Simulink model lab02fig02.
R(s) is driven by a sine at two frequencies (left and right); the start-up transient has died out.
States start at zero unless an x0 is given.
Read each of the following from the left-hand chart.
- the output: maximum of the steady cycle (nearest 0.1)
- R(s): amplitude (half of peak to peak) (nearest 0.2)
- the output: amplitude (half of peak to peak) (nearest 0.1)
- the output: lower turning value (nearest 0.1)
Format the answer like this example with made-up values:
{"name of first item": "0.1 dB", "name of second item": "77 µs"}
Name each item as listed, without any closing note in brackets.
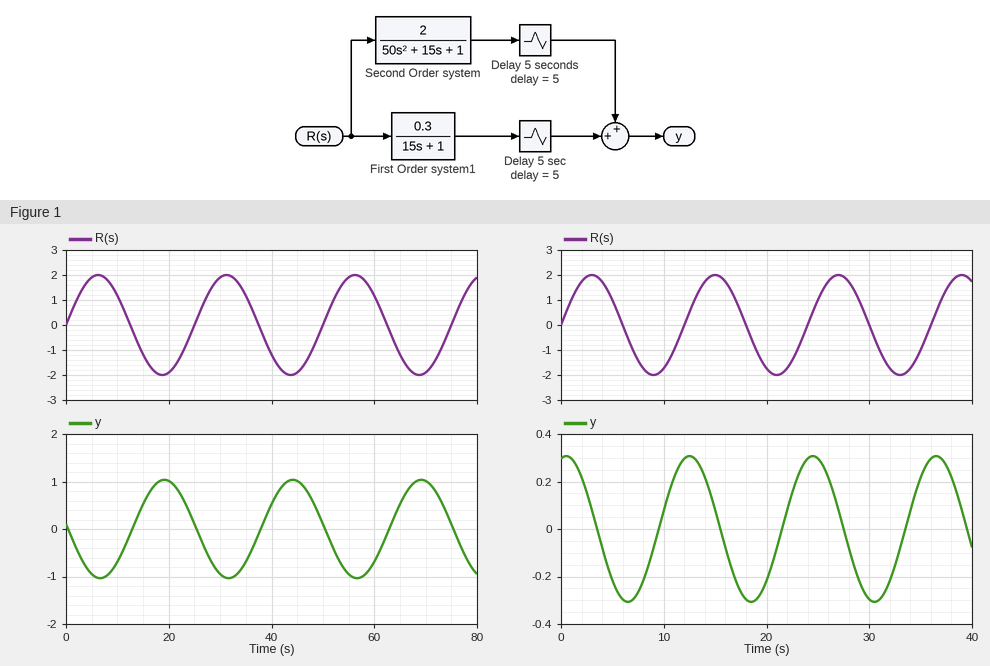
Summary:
{"the output: maximum of the steady cycle": "1.0", "R(s): amplitude (half of peak to peak)": "2.0", "the output: amplitude (half of peak to peak)": "1.0", "the output: lower turning value": "-1.0"}
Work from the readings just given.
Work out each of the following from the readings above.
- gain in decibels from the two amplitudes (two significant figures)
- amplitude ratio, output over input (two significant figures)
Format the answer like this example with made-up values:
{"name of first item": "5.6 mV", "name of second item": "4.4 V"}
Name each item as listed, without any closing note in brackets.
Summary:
{"gain in decibels from the two amplitudes": "-6.0 dB", "amplitude ratio, output over input": "0.50"}
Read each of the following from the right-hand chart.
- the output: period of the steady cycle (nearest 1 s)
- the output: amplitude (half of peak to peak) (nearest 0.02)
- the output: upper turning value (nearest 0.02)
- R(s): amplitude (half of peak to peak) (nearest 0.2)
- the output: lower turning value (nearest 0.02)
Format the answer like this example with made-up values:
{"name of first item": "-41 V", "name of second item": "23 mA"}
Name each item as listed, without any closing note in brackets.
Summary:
{"the output: period of the steady cycle": "12 s", "the output: amplitude (half of peak to peak)": "0.30", "the output: upper turning value": "0.30", "R(s): amplitude (half of peak to peak)": "2.0", "the output: lower turning value": "-0.30"}
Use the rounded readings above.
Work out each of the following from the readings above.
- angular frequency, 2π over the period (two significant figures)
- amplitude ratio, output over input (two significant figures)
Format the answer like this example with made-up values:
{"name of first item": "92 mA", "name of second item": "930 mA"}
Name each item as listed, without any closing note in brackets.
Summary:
{"angular frequency, 2π over the period": "0.52 rad/s", "amplitude ratio, output over input": "0.15"}
